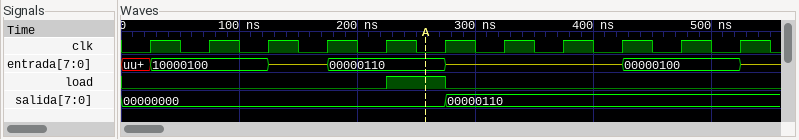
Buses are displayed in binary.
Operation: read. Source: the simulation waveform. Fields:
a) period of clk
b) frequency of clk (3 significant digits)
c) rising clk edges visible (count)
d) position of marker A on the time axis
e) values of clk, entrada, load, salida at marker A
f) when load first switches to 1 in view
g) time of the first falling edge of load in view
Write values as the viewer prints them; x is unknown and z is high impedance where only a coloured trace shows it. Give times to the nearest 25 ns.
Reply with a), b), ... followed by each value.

a) 50 ns
b) 20.0 MHz
c) 11
d) 250 ns
e) clk=0, entrada=00000110, load=1, salida=00000000
f) 225 ns
g) 275 ns
